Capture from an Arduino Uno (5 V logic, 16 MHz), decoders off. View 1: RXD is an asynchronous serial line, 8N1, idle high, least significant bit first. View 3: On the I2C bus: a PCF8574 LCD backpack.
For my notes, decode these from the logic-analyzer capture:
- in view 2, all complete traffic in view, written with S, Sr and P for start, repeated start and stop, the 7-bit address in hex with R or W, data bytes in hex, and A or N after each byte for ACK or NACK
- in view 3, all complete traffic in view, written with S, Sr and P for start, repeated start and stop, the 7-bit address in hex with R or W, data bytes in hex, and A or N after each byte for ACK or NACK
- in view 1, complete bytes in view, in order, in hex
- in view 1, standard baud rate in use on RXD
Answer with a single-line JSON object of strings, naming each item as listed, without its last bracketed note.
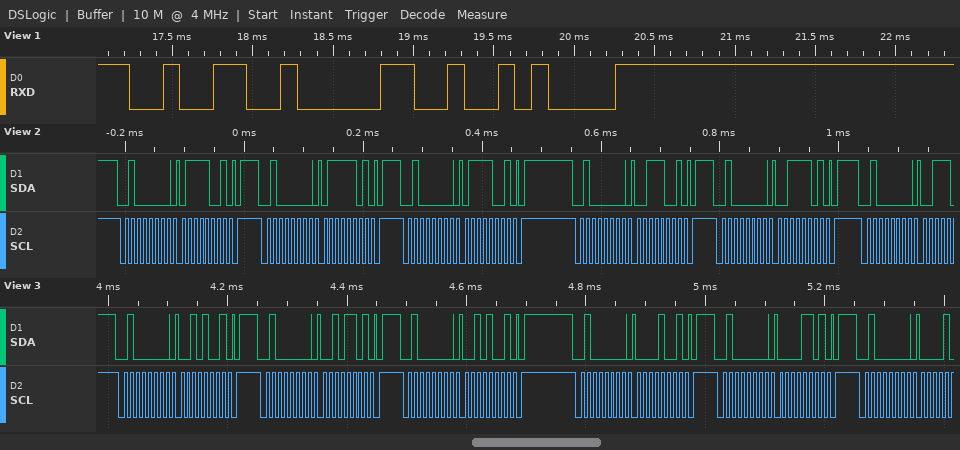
{"in view 2, all complete traffic in view, written with S, Sr and P for start, repeated start and stop, the 7-bit address in hex with R or W, data bytes in hex, and A or N after each byte for ACK or NACK": "S 20W A 79 A P S 20W A 7D A P S 20W A 79 A P S 20W A 39 A P S 20W A 3D A P S 20W A", "in view 3, all complete traffic in view, written with S, Sr and P for start, repeated start and stop, the 7-bit address in hex with R or W, data bytes in hex, and A or N after each byte for ACK or NACK": "S 20W A 29 A P S 20W A 2D A P S 20W A 29 A P S 20W A 09 A P S 20W A 0D A P S 20W A", "in view 1, complete bytes in view, in order, in hex": "32 30 0A", "in view 1, standard baud rate in use on RXD": "9600 baud"}
